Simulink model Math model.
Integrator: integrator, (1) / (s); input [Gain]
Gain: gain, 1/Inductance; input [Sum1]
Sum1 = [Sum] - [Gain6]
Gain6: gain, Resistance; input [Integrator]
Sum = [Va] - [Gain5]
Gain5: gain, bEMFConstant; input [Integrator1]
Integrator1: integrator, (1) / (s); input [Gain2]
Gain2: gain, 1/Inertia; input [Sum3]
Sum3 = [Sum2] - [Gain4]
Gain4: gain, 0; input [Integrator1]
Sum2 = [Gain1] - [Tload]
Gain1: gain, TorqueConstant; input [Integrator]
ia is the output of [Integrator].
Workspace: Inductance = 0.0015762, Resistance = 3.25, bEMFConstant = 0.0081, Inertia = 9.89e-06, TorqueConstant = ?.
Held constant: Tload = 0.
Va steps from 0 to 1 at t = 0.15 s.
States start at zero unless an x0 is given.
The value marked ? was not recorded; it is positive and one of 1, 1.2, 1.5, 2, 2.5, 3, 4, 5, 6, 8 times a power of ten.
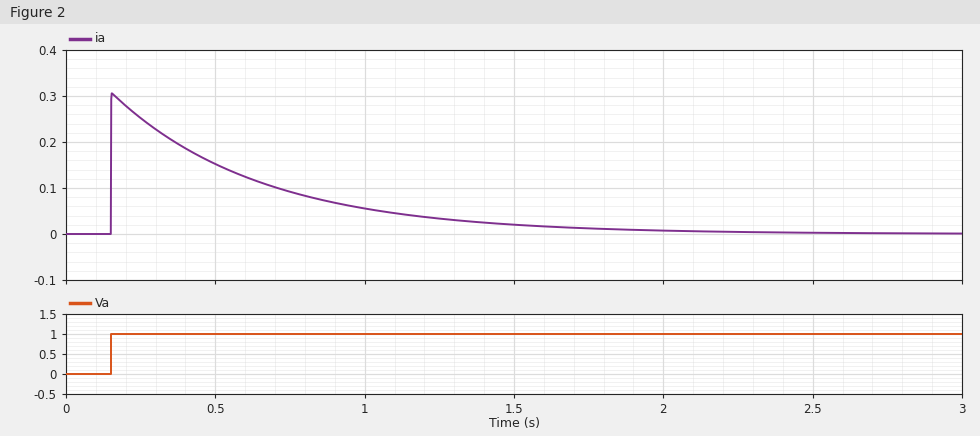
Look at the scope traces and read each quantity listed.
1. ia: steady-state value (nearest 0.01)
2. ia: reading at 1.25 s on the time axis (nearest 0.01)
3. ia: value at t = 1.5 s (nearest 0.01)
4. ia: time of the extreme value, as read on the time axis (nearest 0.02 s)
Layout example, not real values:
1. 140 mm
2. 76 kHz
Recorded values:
1. 0.00
2. 0.03
3. 0.02
4. 0.16 s
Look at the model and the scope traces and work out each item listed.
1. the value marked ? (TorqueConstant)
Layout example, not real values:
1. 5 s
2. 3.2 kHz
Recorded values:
1. 0.008
